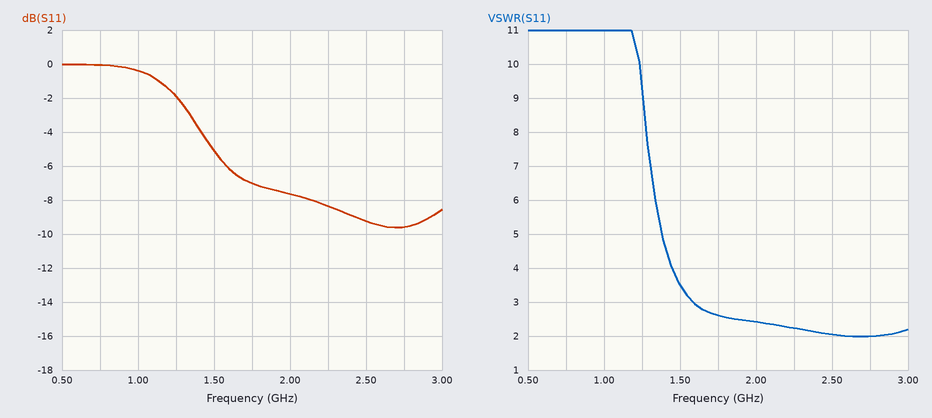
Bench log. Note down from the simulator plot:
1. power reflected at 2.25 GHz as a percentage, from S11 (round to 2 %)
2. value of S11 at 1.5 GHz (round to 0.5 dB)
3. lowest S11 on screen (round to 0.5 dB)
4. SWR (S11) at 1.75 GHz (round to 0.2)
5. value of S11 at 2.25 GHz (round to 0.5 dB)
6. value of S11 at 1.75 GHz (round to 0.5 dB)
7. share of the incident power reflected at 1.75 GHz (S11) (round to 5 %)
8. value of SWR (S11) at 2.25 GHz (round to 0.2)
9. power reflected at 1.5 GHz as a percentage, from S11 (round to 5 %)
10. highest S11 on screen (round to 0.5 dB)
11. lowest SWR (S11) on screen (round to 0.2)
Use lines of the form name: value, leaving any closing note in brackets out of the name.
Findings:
power reflected at 2.25 GHz as a percentage, from S11: 14 %
value of S11 at 1.5 GHz: -5.0 dB
lowest S11 on screen: -9.5 dB
SWR (S11) at 1.75 GHz: 2.6
value of S11 at 2.25 GHz: -8.5 dB
value of S11 at 1.75 GHz: -7.0 dB
share of the incident power reflected at 1.75 GHz (S11): 20 %
value of SWR (S11) at 2.25 GHz: 2.2
power reflected at 1.5 GHz as a percentage, from S11: 30 %
highest S11 on screen: 0.0 dB
lowest SWR (S11) on screen: 2.0
